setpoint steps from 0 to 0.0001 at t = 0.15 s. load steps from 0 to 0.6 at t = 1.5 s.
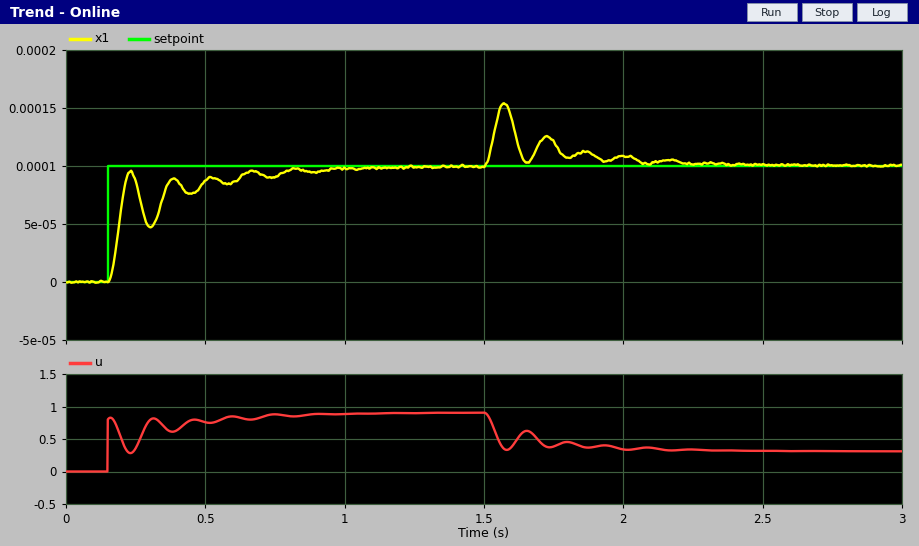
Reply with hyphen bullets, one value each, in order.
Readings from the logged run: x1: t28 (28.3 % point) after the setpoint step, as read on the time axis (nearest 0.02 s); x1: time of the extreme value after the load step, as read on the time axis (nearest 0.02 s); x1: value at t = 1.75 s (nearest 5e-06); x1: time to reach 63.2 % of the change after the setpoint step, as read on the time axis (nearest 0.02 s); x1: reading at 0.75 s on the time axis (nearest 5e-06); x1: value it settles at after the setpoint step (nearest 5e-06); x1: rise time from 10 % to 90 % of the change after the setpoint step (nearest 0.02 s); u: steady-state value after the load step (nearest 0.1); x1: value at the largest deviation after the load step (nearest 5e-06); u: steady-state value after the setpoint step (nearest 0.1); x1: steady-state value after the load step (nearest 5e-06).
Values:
- 0.18 s
- 1.58 s
- 0.000120
- 0.20 s
- 0.000090
- 0.000100
- 0.06 s
- 0.3
- 0.000155
- 0.9
- 0.000100
